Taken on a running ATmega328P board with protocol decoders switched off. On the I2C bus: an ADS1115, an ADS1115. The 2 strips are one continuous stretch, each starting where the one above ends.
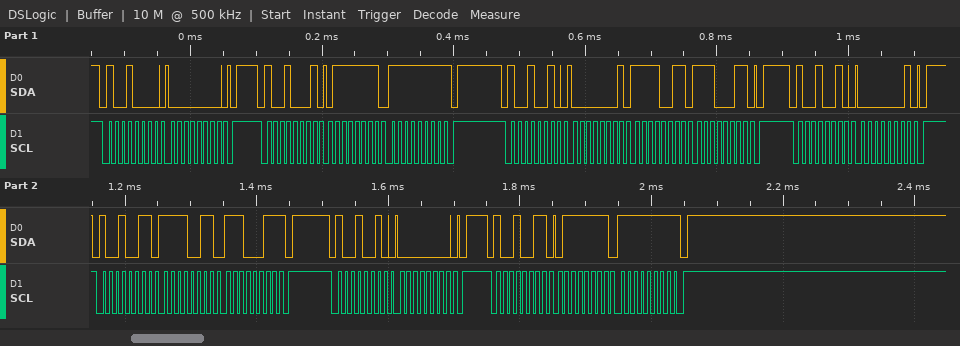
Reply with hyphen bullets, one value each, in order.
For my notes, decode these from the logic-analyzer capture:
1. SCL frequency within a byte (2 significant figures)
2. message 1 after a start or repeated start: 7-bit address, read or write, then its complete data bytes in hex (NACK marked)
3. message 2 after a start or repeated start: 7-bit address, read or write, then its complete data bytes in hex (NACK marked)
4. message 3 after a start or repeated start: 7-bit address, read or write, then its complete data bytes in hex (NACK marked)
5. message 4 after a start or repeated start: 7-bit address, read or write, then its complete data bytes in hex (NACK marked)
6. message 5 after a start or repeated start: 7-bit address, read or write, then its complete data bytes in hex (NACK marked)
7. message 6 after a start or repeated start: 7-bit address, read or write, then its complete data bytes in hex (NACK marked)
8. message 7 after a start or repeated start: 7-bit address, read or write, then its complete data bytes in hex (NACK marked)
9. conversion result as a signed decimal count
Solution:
- 100 kHz
- 0x48 write: 00
- 0x48 read: 7F FF NACK
- 0x49 write: 01 F3 E3
- 0x49 write: 01
- 0x49 read: F3 E3 NACK
- 0x49 write: 00
- 0x49 read: 7F FF NACK
- 32767
